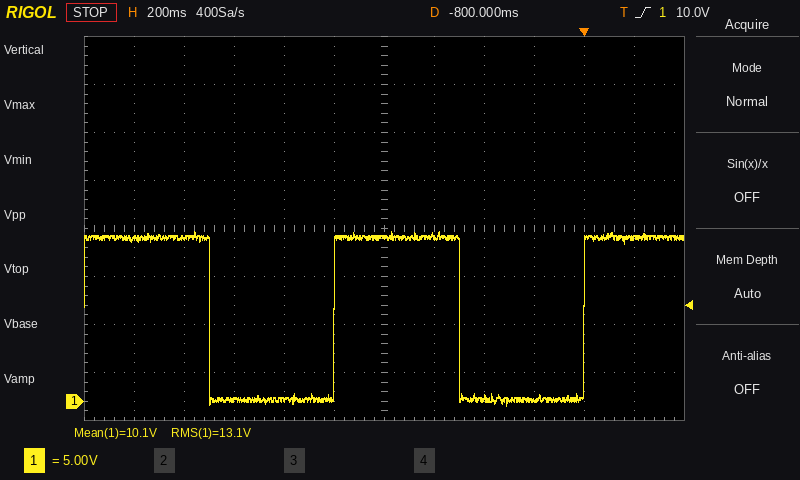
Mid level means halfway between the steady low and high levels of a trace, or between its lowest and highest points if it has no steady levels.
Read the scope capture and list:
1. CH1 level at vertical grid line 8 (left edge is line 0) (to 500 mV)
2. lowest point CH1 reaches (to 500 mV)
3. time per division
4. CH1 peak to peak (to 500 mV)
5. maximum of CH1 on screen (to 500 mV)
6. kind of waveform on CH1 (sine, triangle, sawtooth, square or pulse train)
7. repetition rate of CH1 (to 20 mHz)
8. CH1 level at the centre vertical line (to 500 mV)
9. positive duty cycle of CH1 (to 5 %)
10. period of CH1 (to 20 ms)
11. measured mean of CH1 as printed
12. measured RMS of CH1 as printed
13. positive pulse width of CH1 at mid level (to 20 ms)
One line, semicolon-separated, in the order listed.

500 mV; -500 mV; 200 ms; 18.0 V; 17.5 V; square; 1.00 Hz; 17.0 V; 50 %; 1.00 s; 10.1 V; 13.1 V; 500 ms
